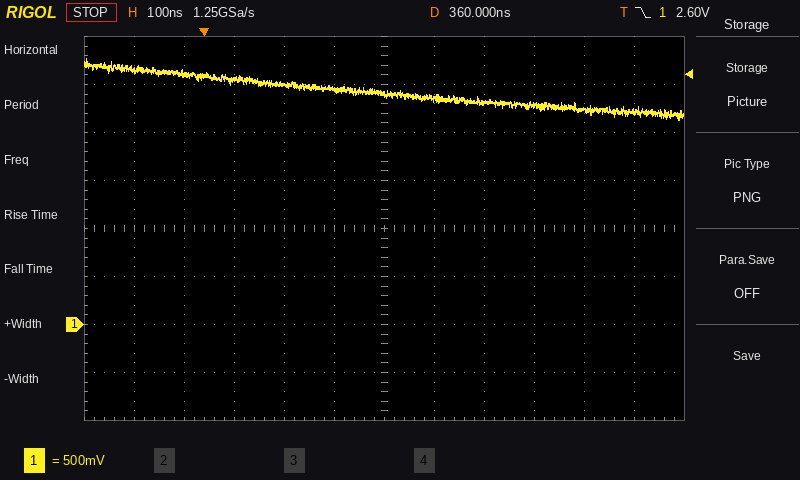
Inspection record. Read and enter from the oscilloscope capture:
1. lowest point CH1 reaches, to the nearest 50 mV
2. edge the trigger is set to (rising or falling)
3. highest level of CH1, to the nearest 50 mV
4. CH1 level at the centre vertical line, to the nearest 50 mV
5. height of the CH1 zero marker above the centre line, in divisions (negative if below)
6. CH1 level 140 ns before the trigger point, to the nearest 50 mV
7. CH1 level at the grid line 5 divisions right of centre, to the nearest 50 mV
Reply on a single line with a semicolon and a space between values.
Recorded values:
2.15 V; falling; 2.75 V; 2.40 V; -2.0 div; 2.65 V; 2.20 V
